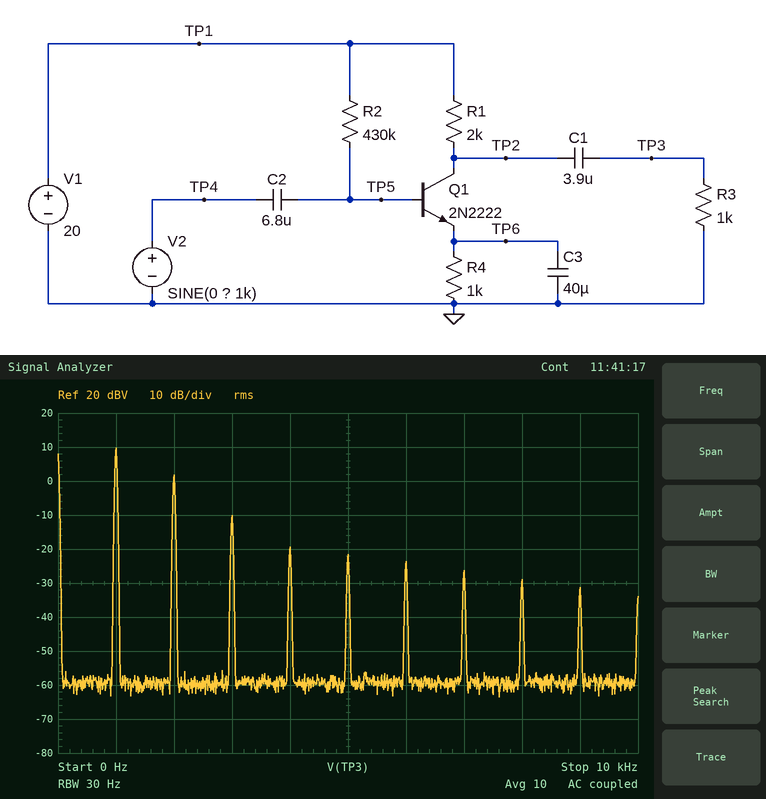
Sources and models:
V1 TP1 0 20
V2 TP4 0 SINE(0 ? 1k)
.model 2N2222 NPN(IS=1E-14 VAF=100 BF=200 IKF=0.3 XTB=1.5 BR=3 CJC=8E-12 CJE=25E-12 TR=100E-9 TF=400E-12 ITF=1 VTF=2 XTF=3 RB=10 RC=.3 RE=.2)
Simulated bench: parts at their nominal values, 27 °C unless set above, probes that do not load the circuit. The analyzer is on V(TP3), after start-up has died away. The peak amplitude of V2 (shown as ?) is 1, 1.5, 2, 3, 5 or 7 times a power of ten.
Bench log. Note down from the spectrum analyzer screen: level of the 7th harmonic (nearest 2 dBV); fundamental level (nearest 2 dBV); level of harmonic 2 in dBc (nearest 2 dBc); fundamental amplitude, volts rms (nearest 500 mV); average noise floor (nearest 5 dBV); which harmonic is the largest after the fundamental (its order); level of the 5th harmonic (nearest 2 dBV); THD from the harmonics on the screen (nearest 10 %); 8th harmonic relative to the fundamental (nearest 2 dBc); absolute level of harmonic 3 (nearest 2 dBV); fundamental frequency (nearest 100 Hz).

-26 dBV
10 dBV
-8 dBc
3.0 V
-60 dBV
2
-22 dBV
40 %
-38 dBc
-10 dBV
1.0 kHz
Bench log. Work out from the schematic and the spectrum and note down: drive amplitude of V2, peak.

70 mV
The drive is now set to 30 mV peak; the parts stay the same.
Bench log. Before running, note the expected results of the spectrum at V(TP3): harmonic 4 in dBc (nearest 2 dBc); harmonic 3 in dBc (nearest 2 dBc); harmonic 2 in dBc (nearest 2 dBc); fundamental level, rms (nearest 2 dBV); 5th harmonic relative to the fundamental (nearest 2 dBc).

-38 dBc
-34 dBc
-16 dBc
6 dBV
-40 dBc
